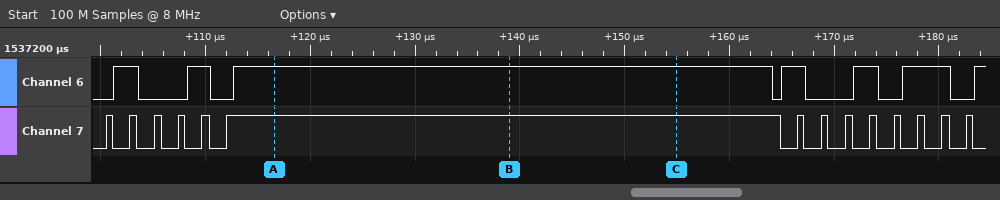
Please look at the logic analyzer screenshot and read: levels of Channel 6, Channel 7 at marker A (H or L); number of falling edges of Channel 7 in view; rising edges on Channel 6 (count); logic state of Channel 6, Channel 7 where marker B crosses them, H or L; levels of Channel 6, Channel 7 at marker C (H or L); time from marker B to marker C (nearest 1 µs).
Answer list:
Channel 6=H, Channel 7=H
14
7
Channel 6=H, Channel 7=H
Channel 6=H, Channel 7=H
16 µs
